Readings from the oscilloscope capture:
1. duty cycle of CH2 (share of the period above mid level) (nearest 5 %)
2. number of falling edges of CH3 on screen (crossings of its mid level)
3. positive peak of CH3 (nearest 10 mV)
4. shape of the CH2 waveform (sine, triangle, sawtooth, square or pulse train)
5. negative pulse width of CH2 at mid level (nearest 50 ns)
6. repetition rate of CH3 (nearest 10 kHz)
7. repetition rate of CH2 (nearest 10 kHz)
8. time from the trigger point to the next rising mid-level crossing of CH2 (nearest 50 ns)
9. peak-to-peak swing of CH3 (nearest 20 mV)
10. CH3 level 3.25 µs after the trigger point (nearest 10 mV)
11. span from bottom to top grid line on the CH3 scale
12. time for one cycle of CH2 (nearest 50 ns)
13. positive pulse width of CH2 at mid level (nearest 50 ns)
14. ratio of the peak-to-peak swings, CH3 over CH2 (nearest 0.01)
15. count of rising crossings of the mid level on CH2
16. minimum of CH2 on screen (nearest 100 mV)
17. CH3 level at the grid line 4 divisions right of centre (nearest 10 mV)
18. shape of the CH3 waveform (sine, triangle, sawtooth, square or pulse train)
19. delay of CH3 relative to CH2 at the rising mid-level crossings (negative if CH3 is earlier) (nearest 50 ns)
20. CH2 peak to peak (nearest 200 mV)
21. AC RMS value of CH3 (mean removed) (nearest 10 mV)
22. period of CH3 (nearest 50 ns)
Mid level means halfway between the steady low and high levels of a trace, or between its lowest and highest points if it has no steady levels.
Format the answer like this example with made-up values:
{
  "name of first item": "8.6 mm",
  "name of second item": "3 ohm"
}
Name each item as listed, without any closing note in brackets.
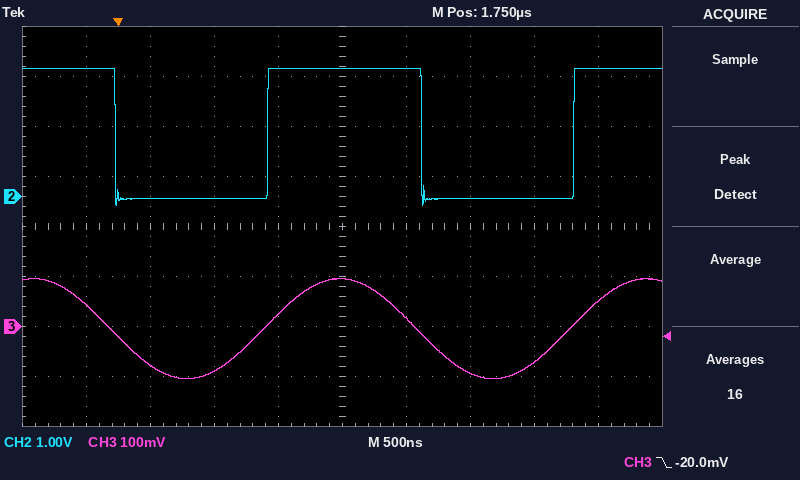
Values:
{
  "duty cycle of CH2 (share of the period above mid level)": "50 %",
  "number of falling edges of CH3 on screen": "2",
  "positive peak of CH3": "100 mV",
  "shape of the CH2 waveform": "square",
  "negative pulse width of CH2 at mid level": "1.20 µs",
  "repetition rate of CH3": "420 kHz",
  "repetition rate of CH2": "420 kHz",
  "time from the trigger point to the next rising mid-level crossing of CH2": "1.15 µs",
  "peak-to-peak swing of CH3": "200 mV",
  "CH3 level 3.25 µs after the trigger point": "-70 mV",
  "span from bottom to top grid line on the CH3 scale": "800 mV",
  "time for one cycle of CH2": "2.40 µs",
  "positive pulse width of CH2 at mid level": "1.20 µs",
  "ratio of the peak-to-peak swings, CH3 over CH2": "0.07",
  "count of rising crossings of the mid level on CH2": "2",
  "minimum of CH2 on screen": "-200 mV",
  "CH3 level at the grid line 4 divisions right of centre": "50 mV",
  "shape of the CH3 waveform": "sine",
  "delay of CH3 relative to CH2 at the rising mid-level crossings (negative if CH3 is earlier)": "-50 ns",
  "CH2 peak to peak": "2.8 V",
  "AC RMS value of CH3 (mean removed)": "70 mV",
  "period of CH3": "2.40 µs"
}
